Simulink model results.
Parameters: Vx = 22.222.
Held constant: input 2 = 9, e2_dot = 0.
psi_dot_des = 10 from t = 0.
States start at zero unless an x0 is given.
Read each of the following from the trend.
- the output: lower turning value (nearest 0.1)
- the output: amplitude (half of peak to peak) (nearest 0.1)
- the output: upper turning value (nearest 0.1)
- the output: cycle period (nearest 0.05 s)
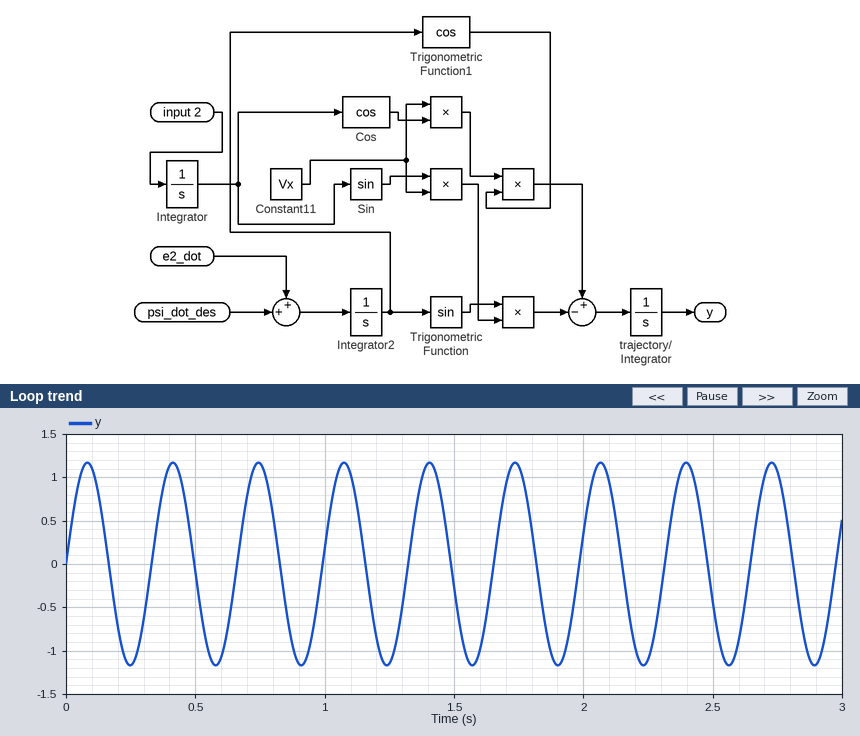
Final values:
-1.2
1.2
1.2
0.35 s
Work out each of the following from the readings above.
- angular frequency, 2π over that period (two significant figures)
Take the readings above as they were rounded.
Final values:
18 rad/s
